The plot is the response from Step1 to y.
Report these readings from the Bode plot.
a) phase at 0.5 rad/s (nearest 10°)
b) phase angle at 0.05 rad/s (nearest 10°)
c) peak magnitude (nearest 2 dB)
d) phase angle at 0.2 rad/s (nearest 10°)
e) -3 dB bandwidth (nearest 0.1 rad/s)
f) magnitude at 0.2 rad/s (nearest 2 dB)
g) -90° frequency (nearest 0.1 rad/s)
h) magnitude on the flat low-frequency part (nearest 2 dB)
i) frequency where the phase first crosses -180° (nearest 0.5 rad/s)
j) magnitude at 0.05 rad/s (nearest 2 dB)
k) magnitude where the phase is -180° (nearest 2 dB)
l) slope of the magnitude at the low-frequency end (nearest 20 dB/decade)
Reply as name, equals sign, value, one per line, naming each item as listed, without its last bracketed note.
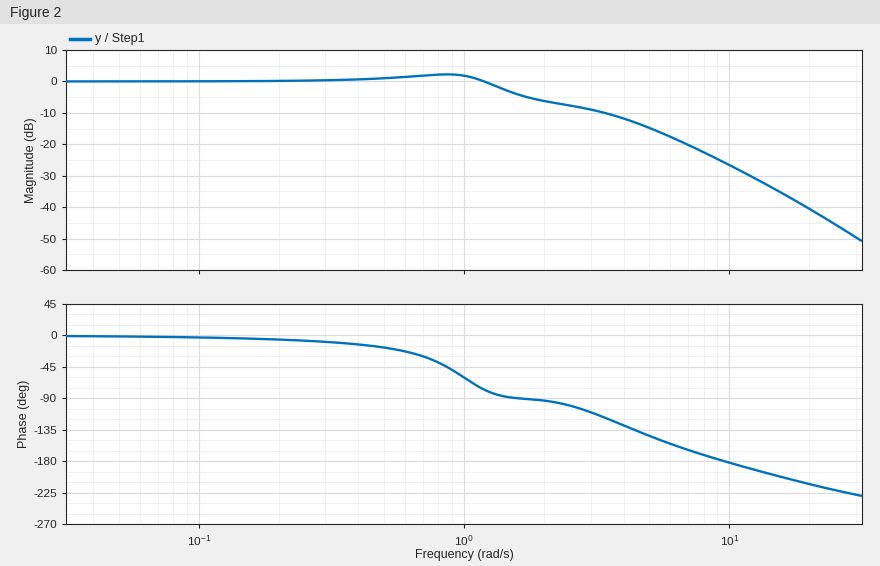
phase at 0.5 rad/s = -20°
phase angle at 0.05 rad/s = 0°
peak magnitude = 2 dB
phase angle at 0.2 rad/s = -10°
-3 dB bandwidth = 1.5 rad/s
magnitude at 0.2 rad/s = 0 dB
-90° frequency = 1.6 rad/s
magnitude on the flat low-frequency part = 0 dB
frequency where the phase first crosses -180° = 9.5 rad/s
magnitude at 0.05 rad/s = 0 dB
magnitude where the phase is -180° = -26 dB
slope of the magnitude at the low-frequency end = 0 dB/decade
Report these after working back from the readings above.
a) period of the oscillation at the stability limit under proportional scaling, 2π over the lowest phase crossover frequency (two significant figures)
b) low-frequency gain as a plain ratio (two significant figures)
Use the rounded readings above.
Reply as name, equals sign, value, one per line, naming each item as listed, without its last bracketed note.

period of the oscillation at the stability limit under proportional scaling, 2π over the lowest phase crossover frequency = 0.66 s
low-frequency gain as a plain ratio = 1.0
